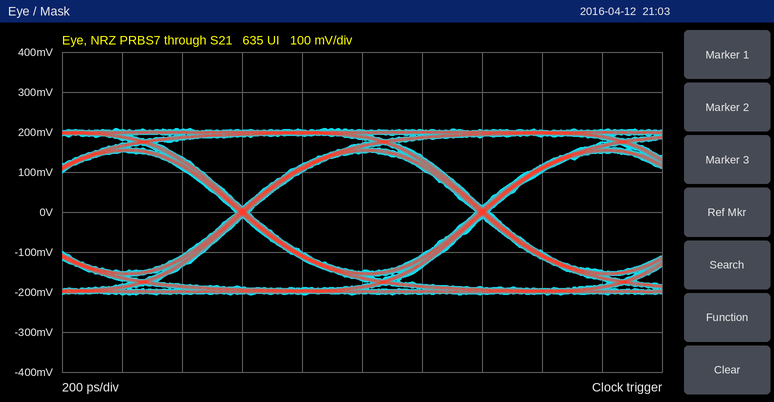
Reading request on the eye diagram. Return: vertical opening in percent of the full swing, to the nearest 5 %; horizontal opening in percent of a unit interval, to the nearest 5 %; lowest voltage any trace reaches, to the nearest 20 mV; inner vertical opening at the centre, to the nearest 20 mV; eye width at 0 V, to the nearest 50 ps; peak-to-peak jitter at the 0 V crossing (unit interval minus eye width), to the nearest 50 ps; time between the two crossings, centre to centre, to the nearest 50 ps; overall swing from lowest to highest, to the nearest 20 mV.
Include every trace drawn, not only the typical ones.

70 %
95 %
-200 mV
300 mV
750 ps
50 ps
800 ps
420 mV
